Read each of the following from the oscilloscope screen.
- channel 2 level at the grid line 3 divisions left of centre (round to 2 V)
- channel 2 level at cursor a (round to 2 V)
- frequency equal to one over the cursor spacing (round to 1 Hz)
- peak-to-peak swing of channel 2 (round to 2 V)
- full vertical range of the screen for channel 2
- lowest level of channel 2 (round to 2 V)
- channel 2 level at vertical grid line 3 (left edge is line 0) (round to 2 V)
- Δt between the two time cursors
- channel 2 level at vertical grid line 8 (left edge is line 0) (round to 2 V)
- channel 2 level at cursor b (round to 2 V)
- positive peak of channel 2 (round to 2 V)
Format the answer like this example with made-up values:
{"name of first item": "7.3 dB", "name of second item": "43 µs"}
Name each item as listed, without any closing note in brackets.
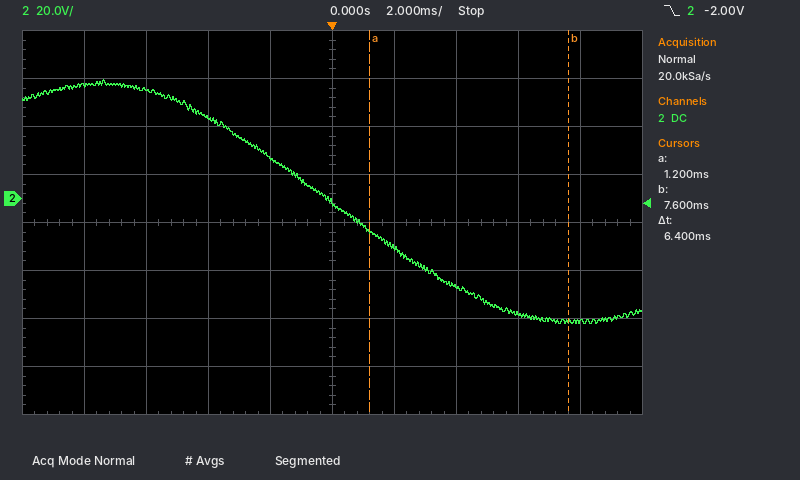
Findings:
{"channel 2 level at the grid line 3 divisions left of centre": "46 V", "channel 2 level at cursor a": "-14 V", "frequency equal to one over the cursor spacing": "156 Hz", "peak-to-peak swing of channel 2": "102 V", "full vertical range of the screen for channel 2": "160 V", "lowest level of channel 2": "-52 V", "channel 2 level at vertical grid line 3 (left edge is line 0)": "34 V", "Δt between the two time cursors": "6.4 ms", "channel 2 level at vertical grid line 8 (left edge is line 0)": "-48 V", "channel 2 level at cursor b": "-52 V", "positive peak of channel 2": "50 V"}
